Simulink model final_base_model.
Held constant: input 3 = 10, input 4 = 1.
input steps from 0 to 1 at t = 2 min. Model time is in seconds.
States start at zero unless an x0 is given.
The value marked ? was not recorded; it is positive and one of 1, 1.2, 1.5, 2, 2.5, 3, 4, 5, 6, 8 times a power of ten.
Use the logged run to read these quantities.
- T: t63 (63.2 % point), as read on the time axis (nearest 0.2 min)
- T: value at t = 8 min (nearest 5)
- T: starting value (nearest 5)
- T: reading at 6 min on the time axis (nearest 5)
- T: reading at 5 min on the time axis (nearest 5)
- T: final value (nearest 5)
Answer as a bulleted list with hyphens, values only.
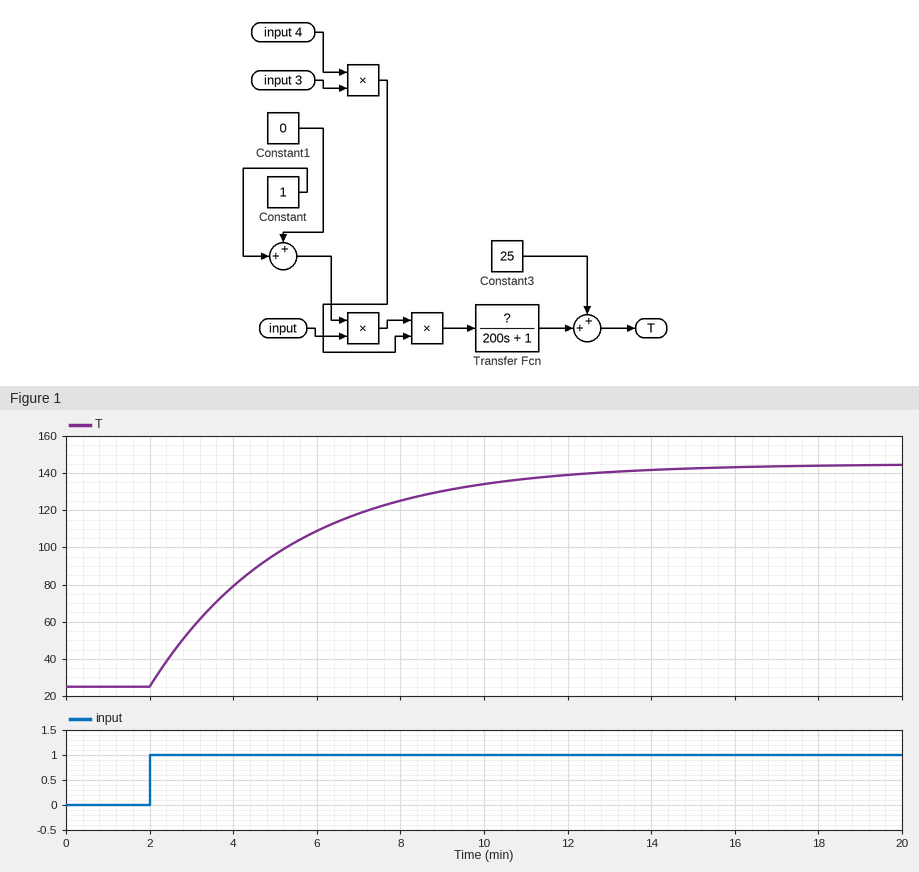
- 5.4 min
- 125
- 25
- 110
- 95
- 145
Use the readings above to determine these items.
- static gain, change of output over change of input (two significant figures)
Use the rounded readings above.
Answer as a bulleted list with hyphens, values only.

- 120
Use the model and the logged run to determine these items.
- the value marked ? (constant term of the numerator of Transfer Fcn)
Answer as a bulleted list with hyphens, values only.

- 12
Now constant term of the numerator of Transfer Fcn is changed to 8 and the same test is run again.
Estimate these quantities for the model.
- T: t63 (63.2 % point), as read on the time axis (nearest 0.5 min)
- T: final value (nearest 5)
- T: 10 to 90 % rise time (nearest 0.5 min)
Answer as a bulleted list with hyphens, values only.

- 5.5 min
- 105
- 7.5 min
